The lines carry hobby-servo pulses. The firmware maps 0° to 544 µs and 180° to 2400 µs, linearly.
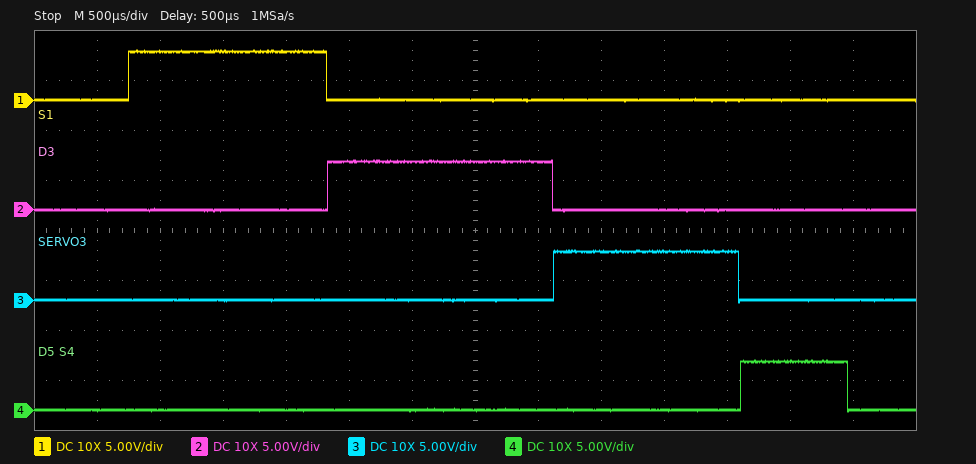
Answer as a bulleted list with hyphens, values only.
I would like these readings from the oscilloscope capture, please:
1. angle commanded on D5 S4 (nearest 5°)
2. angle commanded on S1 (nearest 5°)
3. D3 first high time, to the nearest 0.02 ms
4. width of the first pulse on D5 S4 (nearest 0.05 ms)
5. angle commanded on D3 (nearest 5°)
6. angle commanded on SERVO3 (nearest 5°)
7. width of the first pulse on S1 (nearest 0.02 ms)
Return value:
- 30°
- 100°
- 1.78 ms
- 0.85 ms
- 120°
- 90°
- 1.58 ms
